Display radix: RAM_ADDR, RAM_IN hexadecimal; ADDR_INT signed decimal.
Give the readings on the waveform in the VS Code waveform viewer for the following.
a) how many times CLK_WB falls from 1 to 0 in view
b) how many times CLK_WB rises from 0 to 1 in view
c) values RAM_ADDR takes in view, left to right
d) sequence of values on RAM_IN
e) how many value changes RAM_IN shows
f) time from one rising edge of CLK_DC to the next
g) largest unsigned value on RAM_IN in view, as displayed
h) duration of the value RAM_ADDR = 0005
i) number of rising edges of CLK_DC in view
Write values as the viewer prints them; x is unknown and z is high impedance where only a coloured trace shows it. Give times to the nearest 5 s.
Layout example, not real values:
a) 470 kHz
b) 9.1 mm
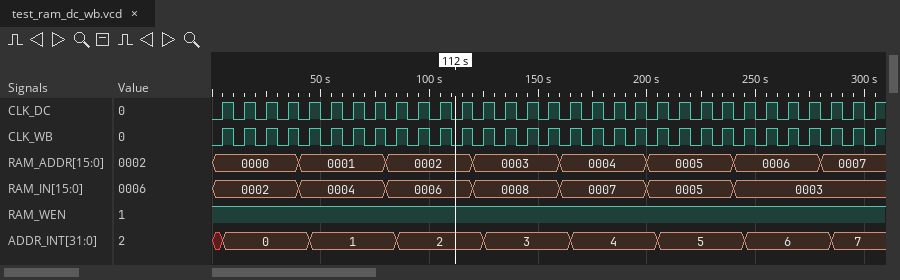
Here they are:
a) 30
b) 31
c) 0000, 0001, 0002, 0003, 0004, 0005, 0006, 0007
d) 0002, 0004, 0006, 0008, 0007, 0005, 0003
e) 6
f) 10 s
g) 0008
h) 40 s
i) 31
